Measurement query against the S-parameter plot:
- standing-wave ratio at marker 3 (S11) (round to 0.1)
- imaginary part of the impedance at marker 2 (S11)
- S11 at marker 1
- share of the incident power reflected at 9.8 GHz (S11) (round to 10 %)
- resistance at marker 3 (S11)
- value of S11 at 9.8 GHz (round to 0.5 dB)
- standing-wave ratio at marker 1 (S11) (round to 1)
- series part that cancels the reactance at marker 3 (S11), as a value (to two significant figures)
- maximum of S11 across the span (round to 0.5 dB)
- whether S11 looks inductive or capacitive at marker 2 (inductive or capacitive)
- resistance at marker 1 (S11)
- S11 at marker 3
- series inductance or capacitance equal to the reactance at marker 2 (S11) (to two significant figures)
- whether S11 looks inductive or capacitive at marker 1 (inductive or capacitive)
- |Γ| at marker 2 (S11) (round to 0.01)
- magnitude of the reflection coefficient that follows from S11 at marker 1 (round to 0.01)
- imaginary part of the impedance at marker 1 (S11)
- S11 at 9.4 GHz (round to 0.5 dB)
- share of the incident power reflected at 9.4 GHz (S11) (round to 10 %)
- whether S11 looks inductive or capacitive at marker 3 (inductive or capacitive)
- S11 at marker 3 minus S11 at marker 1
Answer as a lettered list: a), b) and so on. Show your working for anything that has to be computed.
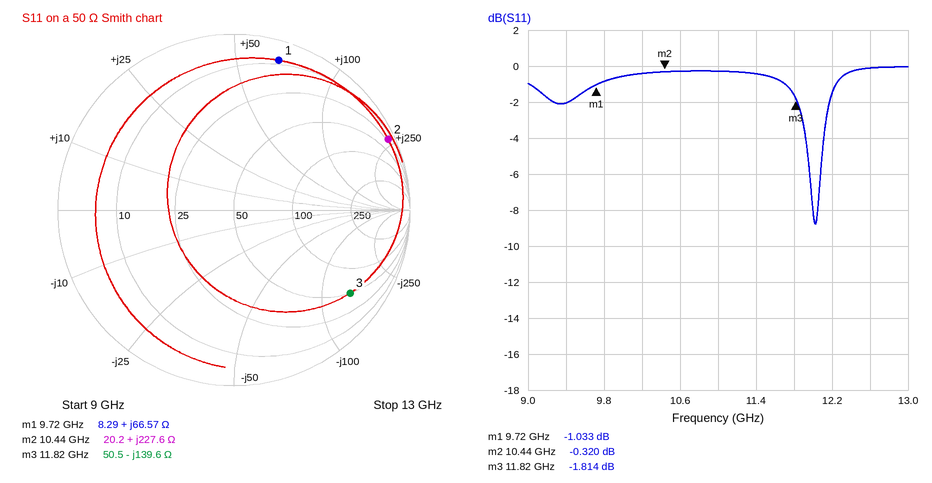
a) 9.6
b) +227.6 Ω
c) -1.033 dB
d) 10^(-1/10) ≈ 79.4 %, so 80 % to the nearest 10 %
e) 50.5 Ω
f) -1.0 dB
g) 17
h) L = 139.6 Ω/(2π × 11.82 GHz) ≈ 1.9 nH
i) 0.0 dB
j) inductive
k) 8.29 Ω
l) -1.814 dB
m) L = 227.6 Ω/(2π × 10.44 GHz) ≈ 3.5 nH
n) inductive
o) 0.96
p) 10^(-1.033/20) ≈ 0.89
q) +66.57 Ω
r) -2.0 dB
s) 10^(-2/10) ≈ 63.1 %, so 60 % to the nearest 10 %
t) capacitive
u) -1.814 − (-1.033) = -0.781 dB
